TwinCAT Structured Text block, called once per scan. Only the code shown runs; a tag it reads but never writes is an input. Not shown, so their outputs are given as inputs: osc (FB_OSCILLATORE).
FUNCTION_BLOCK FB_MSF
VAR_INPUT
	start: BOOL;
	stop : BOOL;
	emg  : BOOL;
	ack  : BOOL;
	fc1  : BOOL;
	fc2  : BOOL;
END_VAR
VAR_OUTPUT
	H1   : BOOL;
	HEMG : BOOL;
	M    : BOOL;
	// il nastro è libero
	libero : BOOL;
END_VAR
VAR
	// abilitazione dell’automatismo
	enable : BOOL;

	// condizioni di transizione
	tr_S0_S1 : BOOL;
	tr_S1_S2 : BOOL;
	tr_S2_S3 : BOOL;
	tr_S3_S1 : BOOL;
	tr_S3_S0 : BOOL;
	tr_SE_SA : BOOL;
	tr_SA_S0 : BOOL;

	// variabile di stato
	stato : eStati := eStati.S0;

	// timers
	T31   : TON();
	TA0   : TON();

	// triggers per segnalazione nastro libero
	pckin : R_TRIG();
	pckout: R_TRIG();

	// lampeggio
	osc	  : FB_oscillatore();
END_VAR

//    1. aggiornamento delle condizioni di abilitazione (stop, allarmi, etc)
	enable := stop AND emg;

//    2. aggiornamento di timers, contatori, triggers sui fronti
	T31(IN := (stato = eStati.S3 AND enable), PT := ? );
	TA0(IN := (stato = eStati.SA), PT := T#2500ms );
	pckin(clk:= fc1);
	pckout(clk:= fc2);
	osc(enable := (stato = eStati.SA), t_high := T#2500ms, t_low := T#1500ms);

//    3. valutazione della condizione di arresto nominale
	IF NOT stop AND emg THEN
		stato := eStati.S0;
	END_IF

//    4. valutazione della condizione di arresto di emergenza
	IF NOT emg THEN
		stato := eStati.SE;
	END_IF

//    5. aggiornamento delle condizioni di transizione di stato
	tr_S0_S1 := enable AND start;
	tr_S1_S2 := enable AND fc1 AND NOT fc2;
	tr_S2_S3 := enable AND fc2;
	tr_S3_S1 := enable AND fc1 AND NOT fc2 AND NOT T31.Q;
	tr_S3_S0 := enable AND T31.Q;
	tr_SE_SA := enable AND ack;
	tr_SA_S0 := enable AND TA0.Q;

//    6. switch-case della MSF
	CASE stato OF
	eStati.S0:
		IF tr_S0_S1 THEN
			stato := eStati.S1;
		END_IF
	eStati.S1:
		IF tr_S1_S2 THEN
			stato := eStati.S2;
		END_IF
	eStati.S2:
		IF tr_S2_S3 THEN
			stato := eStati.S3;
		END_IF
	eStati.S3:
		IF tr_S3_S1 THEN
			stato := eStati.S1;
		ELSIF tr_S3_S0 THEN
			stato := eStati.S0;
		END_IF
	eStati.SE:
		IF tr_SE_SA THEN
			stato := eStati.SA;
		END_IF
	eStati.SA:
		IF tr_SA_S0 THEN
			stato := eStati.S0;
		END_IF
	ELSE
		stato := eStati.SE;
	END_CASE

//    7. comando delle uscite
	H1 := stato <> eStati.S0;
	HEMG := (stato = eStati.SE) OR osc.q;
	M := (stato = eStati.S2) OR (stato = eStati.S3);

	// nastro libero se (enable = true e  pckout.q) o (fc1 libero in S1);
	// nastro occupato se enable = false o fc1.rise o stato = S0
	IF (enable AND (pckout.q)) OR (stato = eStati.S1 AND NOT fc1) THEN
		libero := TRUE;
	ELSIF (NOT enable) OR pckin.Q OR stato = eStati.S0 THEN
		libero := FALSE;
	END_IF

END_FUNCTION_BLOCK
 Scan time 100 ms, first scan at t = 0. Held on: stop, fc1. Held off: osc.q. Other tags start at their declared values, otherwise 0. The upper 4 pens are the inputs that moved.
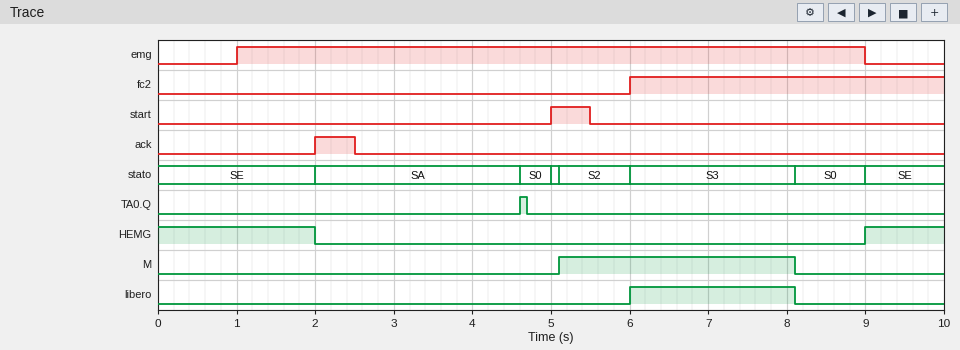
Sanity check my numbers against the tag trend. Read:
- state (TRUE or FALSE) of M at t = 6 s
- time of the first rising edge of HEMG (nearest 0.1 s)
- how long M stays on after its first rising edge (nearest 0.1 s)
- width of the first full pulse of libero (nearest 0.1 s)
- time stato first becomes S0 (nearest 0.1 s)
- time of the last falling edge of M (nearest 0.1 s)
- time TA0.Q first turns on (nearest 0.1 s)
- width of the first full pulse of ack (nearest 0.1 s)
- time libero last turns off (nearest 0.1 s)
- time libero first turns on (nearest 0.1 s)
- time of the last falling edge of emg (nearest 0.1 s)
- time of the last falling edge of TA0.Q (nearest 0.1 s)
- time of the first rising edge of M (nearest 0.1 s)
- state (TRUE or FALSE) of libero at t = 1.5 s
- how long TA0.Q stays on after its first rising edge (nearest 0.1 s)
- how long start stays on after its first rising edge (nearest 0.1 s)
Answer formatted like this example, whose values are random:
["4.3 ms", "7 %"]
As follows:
["TRUE", "9.0 s", "3.0 s", "2.1 s", "4.6 s", "8.1 s", "4.6 s", "0.5 s", "8.1 s", "6.0 s", "9.0 s", "4.7 s", "5.1 s", "FALSE", "0.1 s", "0.5 s"]
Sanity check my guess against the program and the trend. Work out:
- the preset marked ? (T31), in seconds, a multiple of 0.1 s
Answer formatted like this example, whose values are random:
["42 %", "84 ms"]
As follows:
["2.0 s"]
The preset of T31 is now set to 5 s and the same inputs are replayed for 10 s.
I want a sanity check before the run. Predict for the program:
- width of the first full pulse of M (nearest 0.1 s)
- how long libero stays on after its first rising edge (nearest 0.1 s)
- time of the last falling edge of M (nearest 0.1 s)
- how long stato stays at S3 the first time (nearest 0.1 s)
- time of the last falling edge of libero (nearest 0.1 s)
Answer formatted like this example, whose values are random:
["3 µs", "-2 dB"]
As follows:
["3.9 s", "3.0 s", "9.0 s", "3.0 s", "9.0 s"]
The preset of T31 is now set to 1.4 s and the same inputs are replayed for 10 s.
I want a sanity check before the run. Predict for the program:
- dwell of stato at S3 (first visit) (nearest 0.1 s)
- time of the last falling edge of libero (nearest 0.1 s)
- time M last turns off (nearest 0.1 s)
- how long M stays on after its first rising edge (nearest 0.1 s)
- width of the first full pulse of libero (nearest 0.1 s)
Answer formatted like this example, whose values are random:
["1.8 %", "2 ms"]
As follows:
["1.5 s", "7.5 s", "7.5 s", "2.4 s", "1.5 s"]
